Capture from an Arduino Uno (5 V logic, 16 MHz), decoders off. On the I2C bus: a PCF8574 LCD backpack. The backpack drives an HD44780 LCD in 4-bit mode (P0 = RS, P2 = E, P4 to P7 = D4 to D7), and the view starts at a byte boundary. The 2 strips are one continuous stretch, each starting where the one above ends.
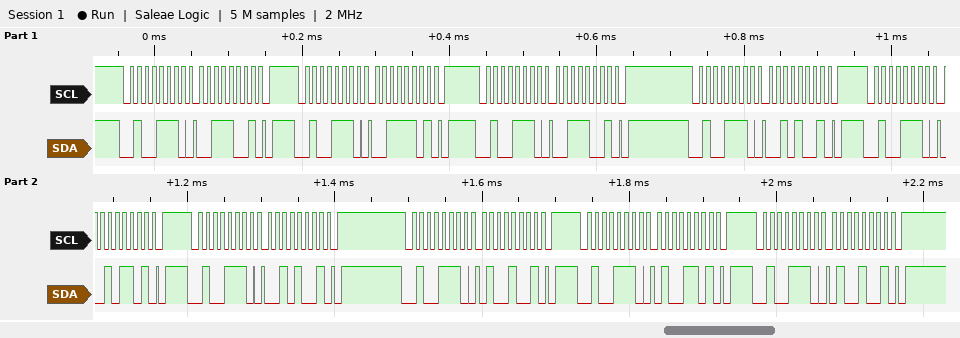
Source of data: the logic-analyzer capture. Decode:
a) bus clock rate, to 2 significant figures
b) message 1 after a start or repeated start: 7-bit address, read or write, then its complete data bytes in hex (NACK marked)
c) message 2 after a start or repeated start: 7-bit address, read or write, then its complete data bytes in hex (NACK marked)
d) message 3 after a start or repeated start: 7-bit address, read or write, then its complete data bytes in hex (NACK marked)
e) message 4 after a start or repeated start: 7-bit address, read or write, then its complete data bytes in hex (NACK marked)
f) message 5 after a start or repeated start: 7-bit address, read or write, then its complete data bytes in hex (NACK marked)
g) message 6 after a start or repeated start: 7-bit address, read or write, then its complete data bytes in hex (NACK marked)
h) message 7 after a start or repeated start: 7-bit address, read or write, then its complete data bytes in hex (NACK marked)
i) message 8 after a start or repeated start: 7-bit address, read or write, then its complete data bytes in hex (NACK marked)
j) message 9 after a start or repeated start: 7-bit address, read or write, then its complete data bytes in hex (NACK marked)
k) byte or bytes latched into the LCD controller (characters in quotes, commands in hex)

100 kHz
0x27 write: 39
0x27 write: 3D
0x27 write: 39
0x27 write: 29
0x27 write: 2D
0x27 write: 29
0x27 write: 49
0x27 write: 4D
0x27 write: 49
'2'
